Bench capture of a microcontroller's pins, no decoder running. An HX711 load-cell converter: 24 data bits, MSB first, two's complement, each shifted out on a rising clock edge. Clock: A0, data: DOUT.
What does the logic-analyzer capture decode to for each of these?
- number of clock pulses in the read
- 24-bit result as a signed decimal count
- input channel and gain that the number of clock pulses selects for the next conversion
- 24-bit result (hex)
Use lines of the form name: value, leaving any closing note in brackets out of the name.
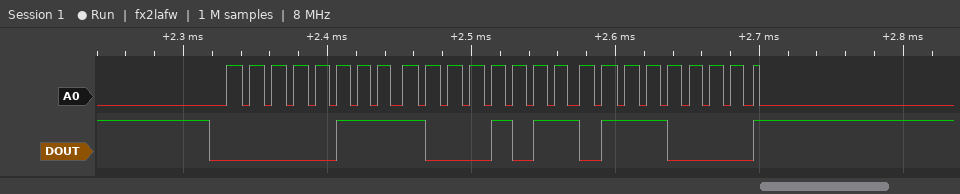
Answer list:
number of clock pulses in the read: 25
24-bit result as a signed decimal count: 494448
input channel and gain that the number of clock pulses selects for the next conversion: channel A, gain 128
24-bit result: 0x078B70
